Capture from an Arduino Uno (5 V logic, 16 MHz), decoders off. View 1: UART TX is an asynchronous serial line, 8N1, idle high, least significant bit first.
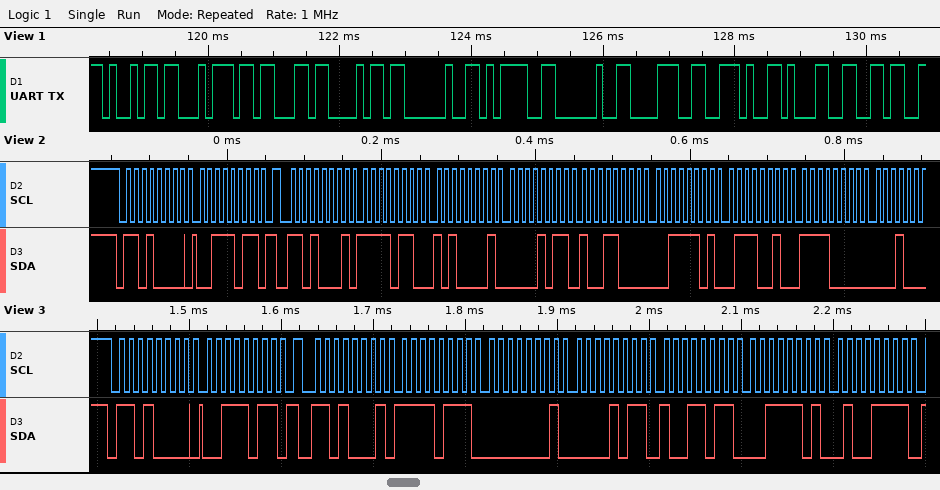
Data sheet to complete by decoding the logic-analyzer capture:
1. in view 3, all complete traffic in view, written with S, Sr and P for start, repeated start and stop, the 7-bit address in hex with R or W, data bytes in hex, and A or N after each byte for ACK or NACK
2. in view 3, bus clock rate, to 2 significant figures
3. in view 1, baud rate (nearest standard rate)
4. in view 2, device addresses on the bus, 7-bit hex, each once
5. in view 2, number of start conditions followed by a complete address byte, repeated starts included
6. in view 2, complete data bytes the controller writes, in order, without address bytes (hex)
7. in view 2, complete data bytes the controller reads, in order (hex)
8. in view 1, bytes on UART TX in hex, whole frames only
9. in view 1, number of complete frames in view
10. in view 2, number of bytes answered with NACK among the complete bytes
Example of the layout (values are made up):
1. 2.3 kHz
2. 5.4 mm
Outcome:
1. S 68W A 3B A Sr 68R A F7 A 01 A 0B A 9B A 3D A 4F A
2. 100 kHz
3. 9600 baud
4. 0x68
5. 2
6. 3B
7. F6 A1 0B 98 3D 72 F0
8. 0x69 0x74 0x63 0x68 0x20 0x3D 0x20 0x38 0x2E 0x31 0x36
9. 11
10. 0
